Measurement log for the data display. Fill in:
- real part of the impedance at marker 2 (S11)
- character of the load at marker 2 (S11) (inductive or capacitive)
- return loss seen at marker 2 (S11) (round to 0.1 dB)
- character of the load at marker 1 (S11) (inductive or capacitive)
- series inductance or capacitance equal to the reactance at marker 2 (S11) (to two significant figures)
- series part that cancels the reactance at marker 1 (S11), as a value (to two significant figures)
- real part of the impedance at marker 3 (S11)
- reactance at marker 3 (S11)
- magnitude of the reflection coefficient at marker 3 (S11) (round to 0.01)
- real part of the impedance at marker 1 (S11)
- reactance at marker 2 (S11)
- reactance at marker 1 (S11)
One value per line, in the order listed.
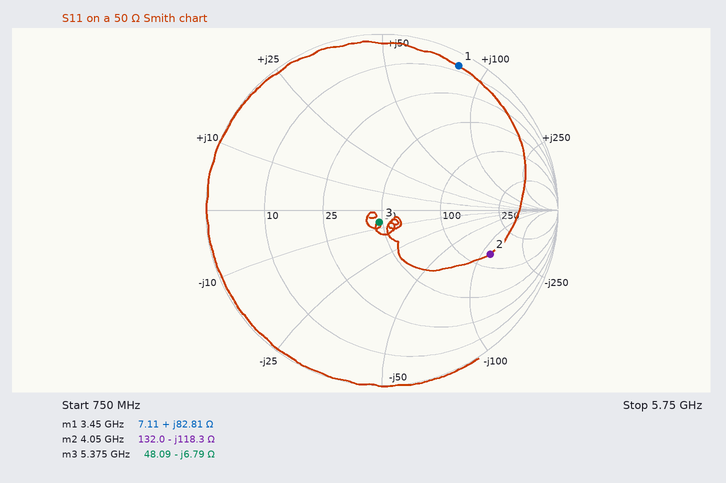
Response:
132.0 Ω
capacitive
3.6 dB
inductive
330 fF
560 fF
48.09 Ω
-6.79 Ω
0.07
7.11 Ω
-118.3 Ω
+82.81 Ω
